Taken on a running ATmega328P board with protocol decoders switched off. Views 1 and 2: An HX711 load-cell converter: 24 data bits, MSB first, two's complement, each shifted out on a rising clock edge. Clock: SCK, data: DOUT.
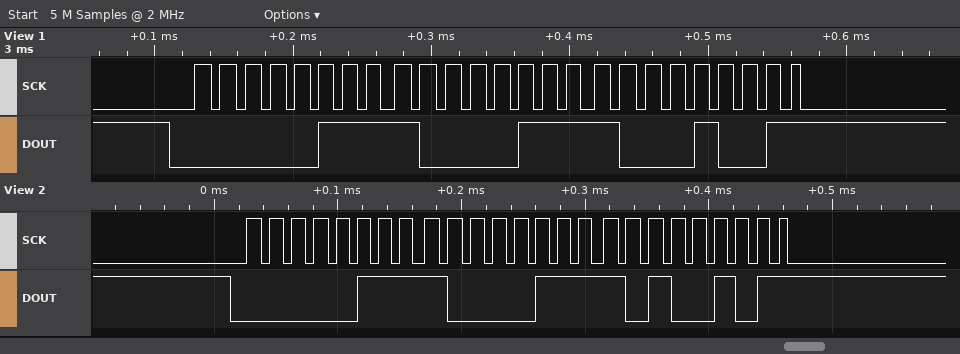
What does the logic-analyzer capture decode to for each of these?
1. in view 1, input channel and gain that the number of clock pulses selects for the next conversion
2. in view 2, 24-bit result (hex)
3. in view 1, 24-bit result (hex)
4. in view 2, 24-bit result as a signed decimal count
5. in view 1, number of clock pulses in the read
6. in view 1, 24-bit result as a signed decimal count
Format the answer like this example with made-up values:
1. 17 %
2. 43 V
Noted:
1. channel A, gain 128
2. 0x0787A5
3. 0x078789
4. 493477
5. 25
6. 493449
